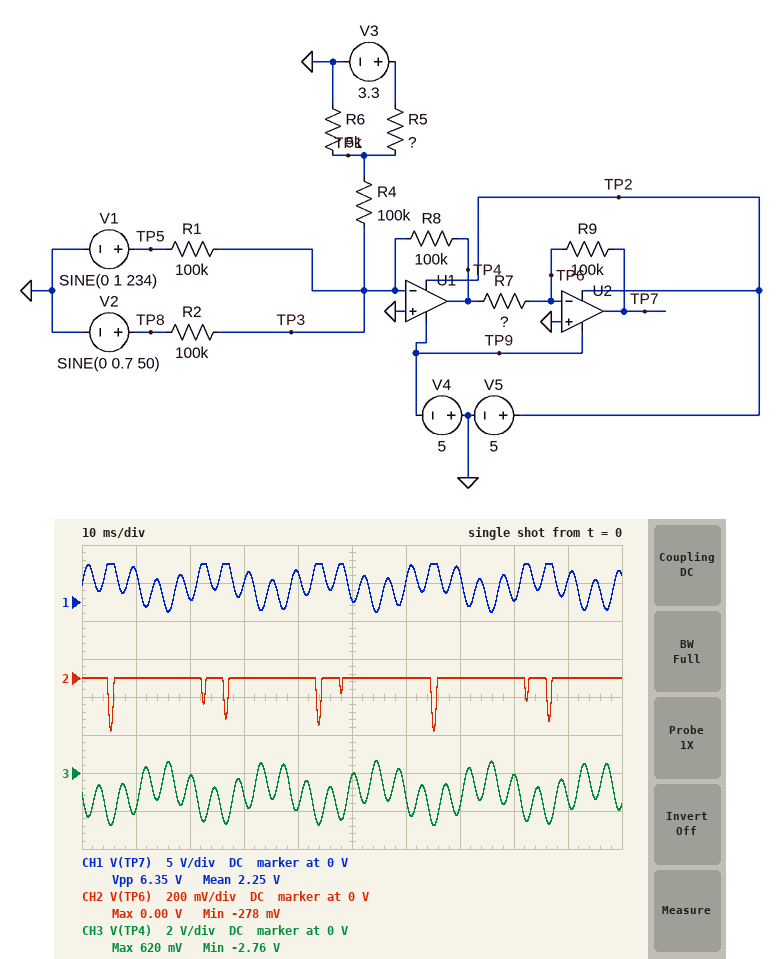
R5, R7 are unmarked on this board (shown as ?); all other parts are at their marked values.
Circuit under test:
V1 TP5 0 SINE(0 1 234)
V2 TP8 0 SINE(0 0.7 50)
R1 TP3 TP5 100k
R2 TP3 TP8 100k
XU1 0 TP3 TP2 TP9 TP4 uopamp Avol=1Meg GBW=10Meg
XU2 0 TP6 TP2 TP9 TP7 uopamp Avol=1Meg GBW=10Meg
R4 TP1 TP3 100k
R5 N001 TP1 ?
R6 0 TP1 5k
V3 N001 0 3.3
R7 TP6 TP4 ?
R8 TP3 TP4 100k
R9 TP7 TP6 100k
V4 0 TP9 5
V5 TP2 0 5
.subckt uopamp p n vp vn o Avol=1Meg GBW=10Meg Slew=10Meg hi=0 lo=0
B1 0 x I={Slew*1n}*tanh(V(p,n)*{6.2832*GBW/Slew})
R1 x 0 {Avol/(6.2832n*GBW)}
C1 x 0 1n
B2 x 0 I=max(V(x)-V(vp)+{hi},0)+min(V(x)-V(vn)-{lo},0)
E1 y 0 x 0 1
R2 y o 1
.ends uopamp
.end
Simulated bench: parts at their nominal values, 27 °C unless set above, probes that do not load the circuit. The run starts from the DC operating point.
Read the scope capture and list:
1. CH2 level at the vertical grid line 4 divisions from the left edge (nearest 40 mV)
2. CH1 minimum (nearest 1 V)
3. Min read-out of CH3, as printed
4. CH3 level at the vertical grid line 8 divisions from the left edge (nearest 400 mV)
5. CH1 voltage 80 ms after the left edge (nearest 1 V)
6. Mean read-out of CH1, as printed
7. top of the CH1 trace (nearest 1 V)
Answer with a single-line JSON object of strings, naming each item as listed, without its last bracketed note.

{"CH2 level at the vertical grid line 4 divisions from the left edge": "0 V", "CH1 minimum": "-1 V", "Min read-out of CH3, as printed": "-2.76 V", "CH3 level at the vertical grid line 8 divisions from the left edge": "0 V", "CH1 voltage 80 ms after the left edge": "0 V", "Mean read-out of CH1, as printed": "2.25 V", "top of the CH1 trace": "5 V"}
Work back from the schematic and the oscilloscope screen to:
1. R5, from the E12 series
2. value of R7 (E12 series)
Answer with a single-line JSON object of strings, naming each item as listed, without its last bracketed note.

{"R5, from the E12 series": "10 kΩ", "value of R7": "47 kΩ"}
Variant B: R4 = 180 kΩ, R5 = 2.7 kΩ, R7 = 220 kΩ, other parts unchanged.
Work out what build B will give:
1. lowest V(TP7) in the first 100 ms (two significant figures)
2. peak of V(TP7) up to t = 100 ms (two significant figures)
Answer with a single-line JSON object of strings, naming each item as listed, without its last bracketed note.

{"lowest V(TP7) in the first 100 ms": "-230 mV", "peak of V(TP7) up to t = 100 ms": "1.3 V"}
